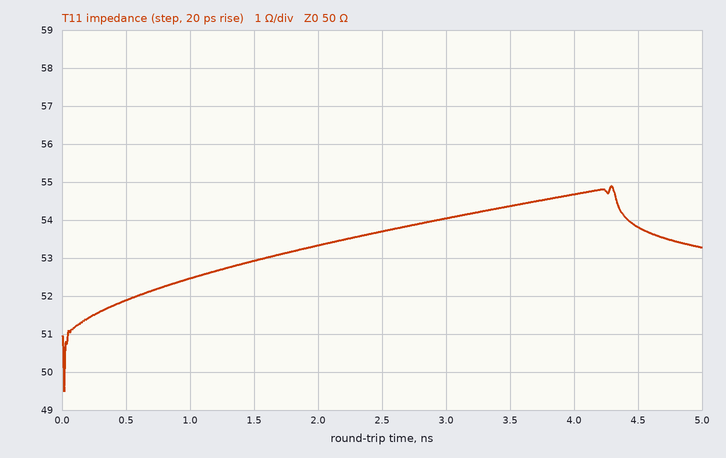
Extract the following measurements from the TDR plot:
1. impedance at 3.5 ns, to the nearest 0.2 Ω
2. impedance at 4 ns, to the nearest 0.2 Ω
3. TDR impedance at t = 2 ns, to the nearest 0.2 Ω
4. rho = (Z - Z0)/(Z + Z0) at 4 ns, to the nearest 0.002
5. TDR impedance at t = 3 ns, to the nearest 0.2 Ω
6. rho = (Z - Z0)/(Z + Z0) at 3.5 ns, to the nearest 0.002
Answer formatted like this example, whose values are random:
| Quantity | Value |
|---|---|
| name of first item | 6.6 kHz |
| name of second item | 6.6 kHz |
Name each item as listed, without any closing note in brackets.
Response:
| Quantity | Value |
|---|---|
| impedance at 3.5 ns, to the nearest 0.2 Ω | 54.4 Ω |
| impedance at 4 ns, to the nearest 0.2 Ω | 54.6 Ω |
| TDR impedance at t = 2 ns, to the nearest 0.2 Ω | 53.4 Ω |
| rho = (Z - Z0)/(Z + Z0) at 4 ns, to the nearest 0.002 | +0.044 |
| TDR impedance at t = 3 ns, to the nearest 0.2 Ω | 54.0 Ω |
| rho = (Z - Z0)/(Z + Z0) at 3.5 ns, to the nearest 0.002 | +0.042 |
